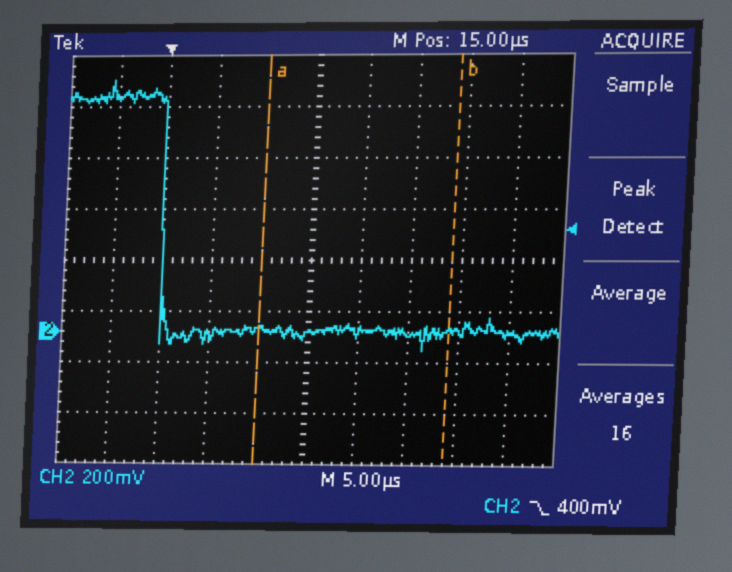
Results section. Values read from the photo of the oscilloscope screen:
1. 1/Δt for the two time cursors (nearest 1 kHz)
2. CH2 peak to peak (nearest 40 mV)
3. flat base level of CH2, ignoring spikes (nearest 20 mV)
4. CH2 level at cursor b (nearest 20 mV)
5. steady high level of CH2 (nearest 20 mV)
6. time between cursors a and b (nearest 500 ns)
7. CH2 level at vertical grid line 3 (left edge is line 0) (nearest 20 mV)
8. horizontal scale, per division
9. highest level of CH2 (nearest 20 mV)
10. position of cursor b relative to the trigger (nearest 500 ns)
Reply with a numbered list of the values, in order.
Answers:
1. 53 kHz
2. 1.04 V
3. 0 mV
4. 0 mV
5. 920 mV
6. 19.0 µs
7. -20 mV
8. 5 µs
9. 980 mV
10. +29.0 µs
